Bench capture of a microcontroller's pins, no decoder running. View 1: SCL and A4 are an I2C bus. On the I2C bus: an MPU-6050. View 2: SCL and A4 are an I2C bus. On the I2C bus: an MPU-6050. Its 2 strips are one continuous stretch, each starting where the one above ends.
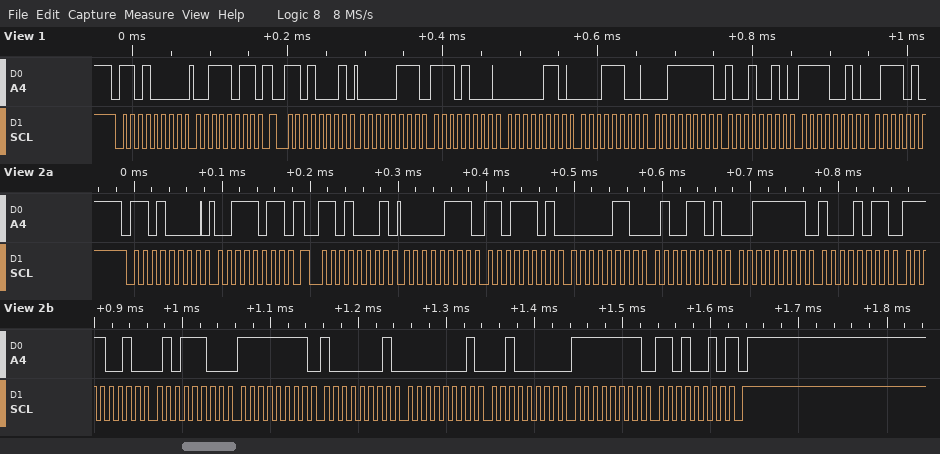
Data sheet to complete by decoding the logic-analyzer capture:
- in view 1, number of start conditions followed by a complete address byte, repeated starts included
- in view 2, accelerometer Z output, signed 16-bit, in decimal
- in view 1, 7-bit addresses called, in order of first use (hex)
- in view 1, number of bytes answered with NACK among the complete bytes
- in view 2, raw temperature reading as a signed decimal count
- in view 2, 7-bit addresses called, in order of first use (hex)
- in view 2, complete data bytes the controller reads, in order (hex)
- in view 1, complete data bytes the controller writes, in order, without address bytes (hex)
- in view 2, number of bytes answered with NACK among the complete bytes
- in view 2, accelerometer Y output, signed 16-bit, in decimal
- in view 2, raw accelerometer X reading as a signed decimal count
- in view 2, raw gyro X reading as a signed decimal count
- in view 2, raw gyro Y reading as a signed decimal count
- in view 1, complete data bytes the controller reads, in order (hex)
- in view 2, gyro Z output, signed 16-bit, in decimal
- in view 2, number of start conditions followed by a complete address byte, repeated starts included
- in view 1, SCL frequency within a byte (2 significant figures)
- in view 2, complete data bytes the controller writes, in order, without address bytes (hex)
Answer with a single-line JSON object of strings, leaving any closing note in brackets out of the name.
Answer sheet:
{"in view 1, number of start conditions followed by a complete address byte, repeated starts included": "2", "in view 2, accelerometer Z output, signed 16-bit, in decimal": "16267", "in view 1, 7-bit addresses called, in order of first use": "0x68", "in view 1, number of bytes answered with NACK among the complete bytes": "0", "in view 2, raw temperature reading as a signed decimal count": "-3492", "in view 2, 7-bit addresses called, in order of first use": "0x68", "in view 2, complete data bytes the controller reads, in order": "07 DD 06 4D 3F 8B F2 5C FF 81 01 20 FF D2", "in view 1, complete data bytes the controller writes, in order, without address bytes": "3B", "in view 2, number of bytes answered with NACK among the complete bytes": "1", "in view 2, accelerometer Y output, signed 16-bit, in decimal": "1613", "in view 2, raw accelerometer X reading as a signed decimal count": "2013", "in view 2, raw gyro X reading as a signed decimal count": "-127", "in view 2, raw gyro Y reading as a signed decimal count": "288", "in view 1, complete data bytes the controller reads, in order": "07 E8 06 1C 3F 92 F2", "in view 2, gyro Z output, signed 16-bit, in decimal": "-46", "in view 2, number of start conditions followed by a complete address byte, repeated starts included": "2", "in view 1, SCL frequency within a byte": "100 kHz", "in view 2, complete data bytes the controller writes, in order, without address bytes": "3B"}
